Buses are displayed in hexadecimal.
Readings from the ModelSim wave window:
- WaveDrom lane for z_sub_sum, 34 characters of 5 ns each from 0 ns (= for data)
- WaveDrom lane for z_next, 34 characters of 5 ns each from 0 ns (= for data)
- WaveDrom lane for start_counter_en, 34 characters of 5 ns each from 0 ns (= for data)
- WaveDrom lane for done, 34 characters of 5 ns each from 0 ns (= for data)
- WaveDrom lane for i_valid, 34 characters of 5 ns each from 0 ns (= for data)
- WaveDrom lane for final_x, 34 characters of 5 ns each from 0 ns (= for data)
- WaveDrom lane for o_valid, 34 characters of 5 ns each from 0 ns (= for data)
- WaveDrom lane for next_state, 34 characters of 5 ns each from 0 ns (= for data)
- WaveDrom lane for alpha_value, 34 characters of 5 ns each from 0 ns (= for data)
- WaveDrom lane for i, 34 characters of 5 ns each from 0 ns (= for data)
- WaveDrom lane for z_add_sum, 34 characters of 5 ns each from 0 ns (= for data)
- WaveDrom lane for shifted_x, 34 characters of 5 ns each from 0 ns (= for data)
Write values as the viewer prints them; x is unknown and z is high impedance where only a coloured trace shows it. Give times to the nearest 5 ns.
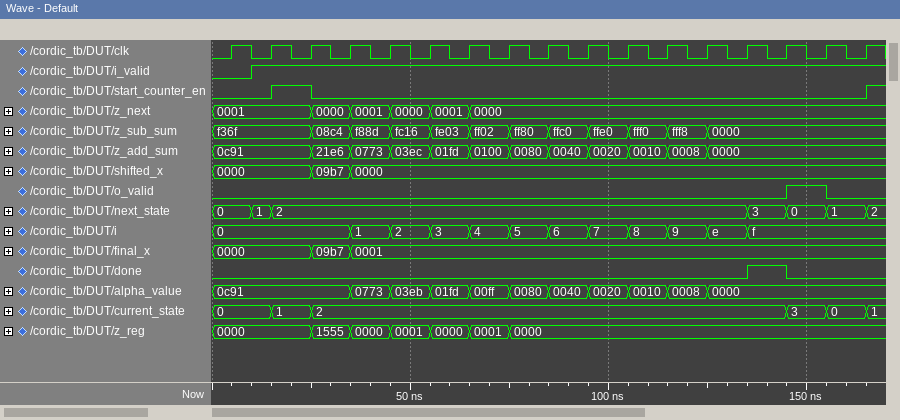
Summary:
{name: 'z_sub_sum', wave: '=....=.=.=.=.=.=.=.=.=.=.=........', data: 'f36f 08c4 f88d fc16 fe03 ff02 ff80 ffc0 ffe0 fff0 fff8 0000'}
{name: 'z_next', wave: '=....=.=.=.=.=....................', data: '0001 0000 0001 0000 0001 0000'}
{name: 'start_counter_en', wave: '0..1.0...........................1'}
{name: 'done', wave: '0..........................1.0....'}
{name: 'i_valid', wave: '0.1...............................'}
{name: 'final_x', wave: '=....=.=..........................', data: '0000 09b7 0001'}
{name: 'o_valid', wave: '0............................1.0..'}
{name: 'next_state', wave: '=.==.......................=.=.=.=', data: '0 1 2 3 0 1 2'}
{name: 'alpha_value', wave: '=......=.=.=.=.=.=.=.=.=.=........', data: '0c91 0773 03eb 01fd 00ff 0080 0040 0020 0010 0008 0000'}
{name: 'i', wave: '=......=.=.=.=.=.=.=.=.=.=.=......', data: '0 1 2 3 4 5 6 7 8 9 e f'}
{name: 'z_add_sum', wave: '=....=.=.=.=.=.=.=.=.=.=.=........', data: '0c91 21e6 0773 03ec 01fd 0100 0080 0040 0020 0010 0008 0000'}
{name: 'shifted_x', wave: '=....=.=..........................', data: '0000 09b7 0000'}
